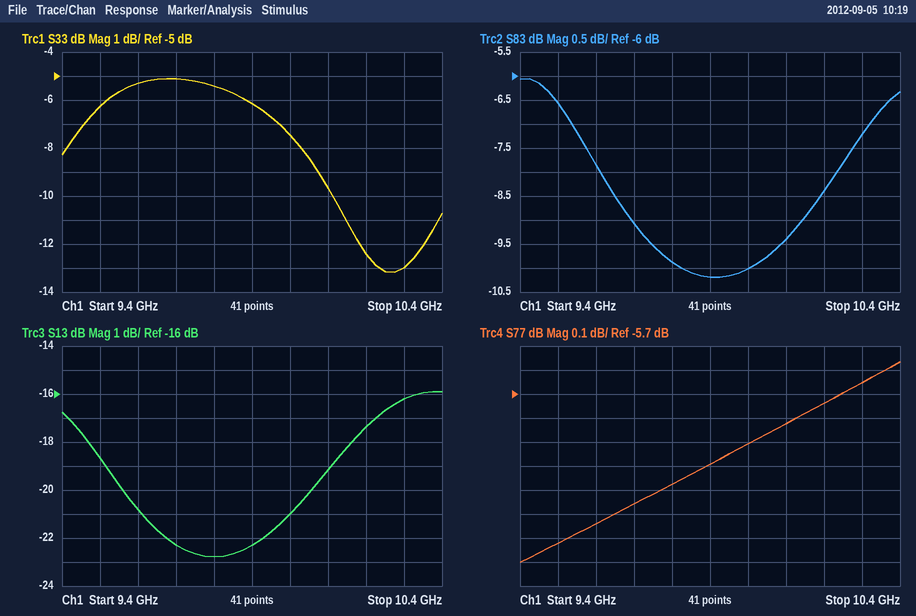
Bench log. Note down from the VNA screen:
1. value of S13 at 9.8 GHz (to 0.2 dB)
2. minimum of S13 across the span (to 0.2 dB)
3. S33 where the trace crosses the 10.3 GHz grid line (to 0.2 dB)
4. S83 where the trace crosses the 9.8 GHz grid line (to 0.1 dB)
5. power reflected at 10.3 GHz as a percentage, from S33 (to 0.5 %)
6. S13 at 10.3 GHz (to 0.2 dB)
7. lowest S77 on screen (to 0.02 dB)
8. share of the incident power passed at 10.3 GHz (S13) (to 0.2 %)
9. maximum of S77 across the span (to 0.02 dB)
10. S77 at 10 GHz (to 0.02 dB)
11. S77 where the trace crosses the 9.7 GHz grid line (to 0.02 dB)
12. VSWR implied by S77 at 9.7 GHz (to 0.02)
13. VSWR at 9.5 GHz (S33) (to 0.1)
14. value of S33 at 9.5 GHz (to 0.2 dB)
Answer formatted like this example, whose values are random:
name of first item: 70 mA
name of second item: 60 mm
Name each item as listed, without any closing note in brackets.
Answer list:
value of S13 at 9.8 GHz: -22.8 dB
minimum of S13 across the span: -22.8 dB
S33 where the trace crosses the 10.3 GHz grid line: -13.0 dB
S83 where the trace crosses the 9.8 GHz grid line: -9.9 dB
power reflected at 10.3 GHz as a percentage, from S33: 5.0 %
S13 at 10.3 GHz: -16.2 dB
lowest S77 on screen: -6.40 dB
share of the incident power passed at 10.3 GHz (S13): 2.4 %
maximum of S77 across the span: -5.56 dB
S77 at 10 GHz: -5.90 dB
S77 where the trace crosses the 9.7 GHz grid line: -6.16 dB
VSWR implied by S77 at 9.7 GHz: 2.94
VSWR at 9.5 GHz (S33): 2.9
value of S33 at 9.5 GHz: -6.2 dB
